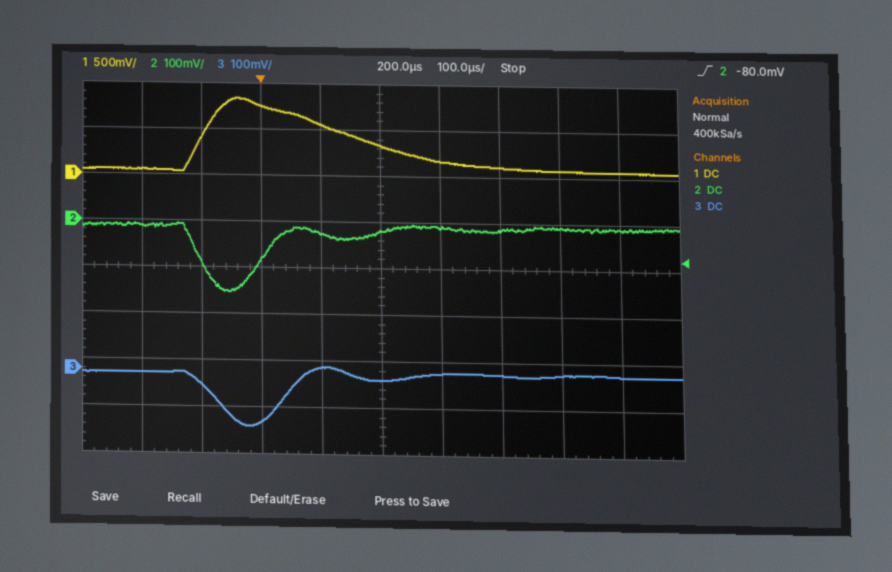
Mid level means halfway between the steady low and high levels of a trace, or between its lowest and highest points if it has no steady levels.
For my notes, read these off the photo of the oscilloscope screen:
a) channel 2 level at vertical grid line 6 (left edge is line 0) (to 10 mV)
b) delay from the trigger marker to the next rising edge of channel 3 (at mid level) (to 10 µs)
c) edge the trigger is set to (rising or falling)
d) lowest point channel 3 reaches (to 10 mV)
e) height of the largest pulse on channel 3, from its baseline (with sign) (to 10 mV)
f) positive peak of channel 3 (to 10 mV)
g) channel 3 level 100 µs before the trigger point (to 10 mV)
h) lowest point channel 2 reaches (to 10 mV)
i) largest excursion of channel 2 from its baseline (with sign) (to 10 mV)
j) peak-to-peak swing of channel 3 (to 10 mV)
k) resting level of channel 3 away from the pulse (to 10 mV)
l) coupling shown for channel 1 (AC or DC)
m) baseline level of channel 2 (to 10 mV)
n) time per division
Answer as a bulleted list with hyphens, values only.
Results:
- -10 mV
- 40 µs
- rising
- -120 mV
- -110 mV
- 10 mV
- -30 mV
- -150 mV
- -140 mV
- 130 mV
- -10 mV
- DC
- -10 mV
- 100 µs
